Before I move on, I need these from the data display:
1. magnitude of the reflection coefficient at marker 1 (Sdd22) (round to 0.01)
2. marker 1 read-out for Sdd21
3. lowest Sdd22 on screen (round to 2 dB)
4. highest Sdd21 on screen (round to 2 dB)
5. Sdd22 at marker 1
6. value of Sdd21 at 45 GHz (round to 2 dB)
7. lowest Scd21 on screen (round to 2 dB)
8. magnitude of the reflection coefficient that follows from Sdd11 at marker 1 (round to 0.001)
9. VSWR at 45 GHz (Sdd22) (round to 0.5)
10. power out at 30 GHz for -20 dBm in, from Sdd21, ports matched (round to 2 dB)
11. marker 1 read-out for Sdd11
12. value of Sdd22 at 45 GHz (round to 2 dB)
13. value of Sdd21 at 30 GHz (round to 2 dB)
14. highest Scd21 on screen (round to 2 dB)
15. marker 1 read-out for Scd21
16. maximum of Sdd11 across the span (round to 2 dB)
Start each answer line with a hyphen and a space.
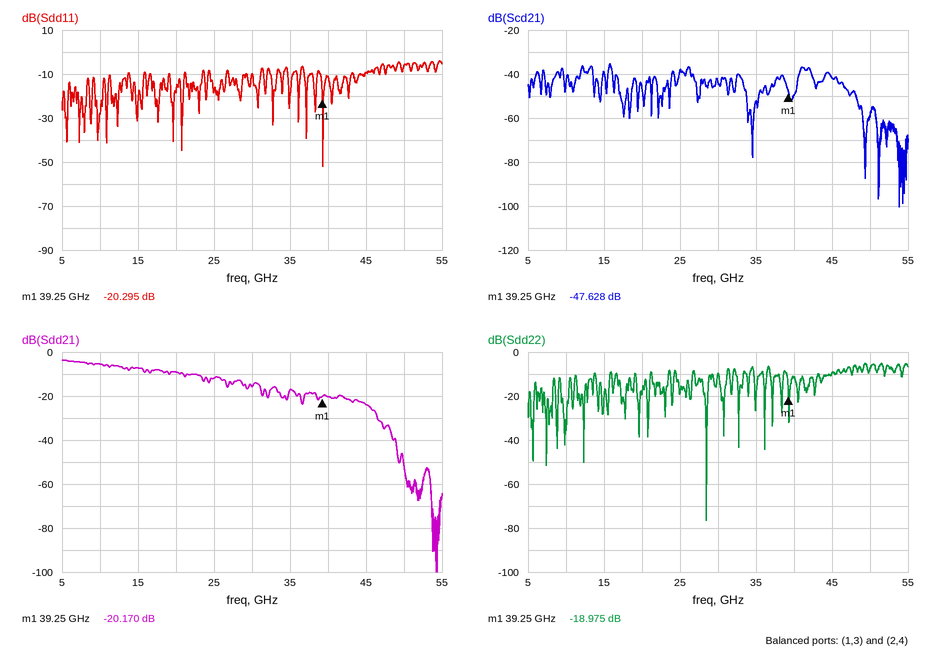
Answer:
- 0.11
- -20.170 dB
- -76 dB
- -4 dB
- -18.975 dB
- -24 dB
- -100 dB
- 0.097
- 2.0
- -36 dBm
- -20.295 dB
- -10 dB
- -16 dB
- -36 dB
- -47.628 dB
- -4 dB
